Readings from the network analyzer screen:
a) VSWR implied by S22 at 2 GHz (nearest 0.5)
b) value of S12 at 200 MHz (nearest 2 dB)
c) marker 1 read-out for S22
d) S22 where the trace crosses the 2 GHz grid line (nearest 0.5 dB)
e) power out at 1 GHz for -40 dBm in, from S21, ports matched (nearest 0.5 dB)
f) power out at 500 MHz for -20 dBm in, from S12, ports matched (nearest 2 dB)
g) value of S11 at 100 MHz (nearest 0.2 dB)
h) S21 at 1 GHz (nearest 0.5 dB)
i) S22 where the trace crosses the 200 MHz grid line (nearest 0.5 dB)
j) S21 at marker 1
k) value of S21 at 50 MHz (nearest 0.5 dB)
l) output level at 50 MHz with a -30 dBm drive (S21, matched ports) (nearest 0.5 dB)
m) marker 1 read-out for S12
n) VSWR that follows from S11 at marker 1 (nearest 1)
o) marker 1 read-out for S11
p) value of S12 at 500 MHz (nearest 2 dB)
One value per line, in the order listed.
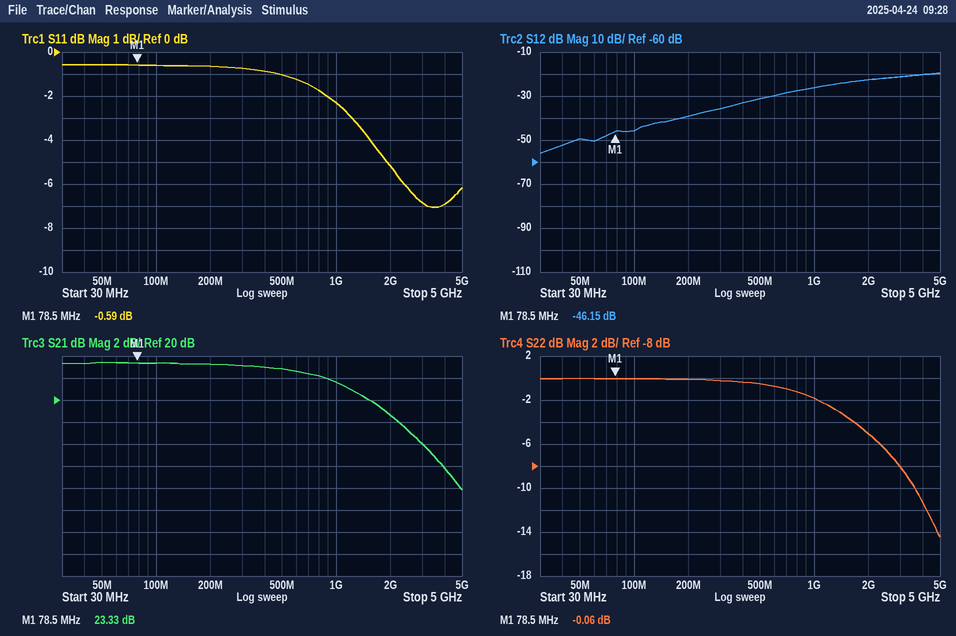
3.5
-40 dB
-0.06 dB
-5.0 dB
-18.5 dBm
-52 dBm
-0.6 dB
21.5 dB
0.0 dB
23.33 dB
23.5 dB
-6.5 dBm
-46.15 dB
29
-0.59 dB
-32 dB
